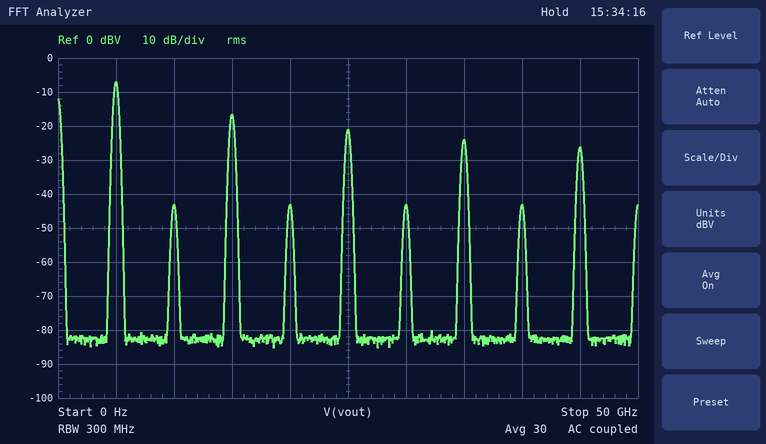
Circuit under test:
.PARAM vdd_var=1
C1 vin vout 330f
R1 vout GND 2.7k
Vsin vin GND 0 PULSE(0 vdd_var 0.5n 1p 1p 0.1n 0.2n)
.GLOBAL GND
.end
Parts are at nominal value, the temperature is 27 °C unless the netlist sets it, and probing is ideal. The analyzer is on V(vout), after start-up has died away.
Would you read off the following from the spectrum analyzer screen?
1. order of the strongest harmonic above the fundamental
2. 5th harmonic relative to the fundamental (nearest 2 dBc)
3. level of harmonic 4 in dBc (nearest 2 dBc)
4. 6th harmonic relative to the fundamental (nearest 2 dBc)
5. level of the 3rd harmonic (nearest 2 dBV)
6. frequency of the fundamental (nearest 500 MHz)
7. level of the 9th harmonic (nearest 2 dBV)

3
-14 dBc
-36 dBc
-36 dBc
-16 dBV
5.0 GHz
-26 dBV
